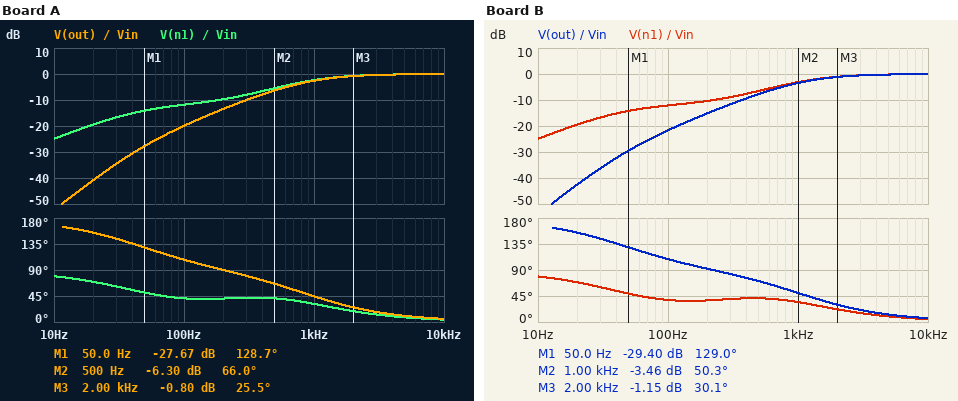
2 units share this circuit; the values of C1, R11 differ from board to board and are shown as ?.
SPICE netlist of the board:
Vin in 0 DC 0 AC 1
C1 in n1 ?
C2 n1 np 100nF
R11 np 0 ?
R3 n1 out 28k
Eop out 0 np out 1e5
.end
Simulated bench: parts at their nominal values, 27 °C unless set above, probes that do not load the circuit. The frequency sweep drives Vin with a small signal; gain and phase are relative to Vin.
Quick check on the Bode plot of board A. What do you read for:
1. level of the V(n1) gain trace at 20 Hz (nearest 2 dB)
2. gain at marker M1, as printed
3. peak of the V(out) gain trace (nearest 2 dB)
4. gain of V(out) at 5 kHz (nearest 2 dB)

-20 dB
-27.67 dB
0 dB
0 dB
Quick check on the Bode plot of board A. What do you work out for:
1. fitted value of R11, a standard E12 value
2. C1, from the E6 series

6.8 kΩ
33 nF
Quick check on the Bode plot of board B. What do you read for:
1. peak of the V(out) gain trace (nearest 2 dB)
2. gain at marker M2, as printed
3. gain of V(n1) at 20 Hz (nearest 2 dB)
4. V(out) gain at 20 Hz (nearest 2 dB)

0 dB
-3.46 dB
-20 dB
-42 dB
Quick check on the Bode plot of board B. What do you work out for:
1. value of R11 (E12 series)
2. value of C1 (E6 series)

5.6 kΩ
33 nF
